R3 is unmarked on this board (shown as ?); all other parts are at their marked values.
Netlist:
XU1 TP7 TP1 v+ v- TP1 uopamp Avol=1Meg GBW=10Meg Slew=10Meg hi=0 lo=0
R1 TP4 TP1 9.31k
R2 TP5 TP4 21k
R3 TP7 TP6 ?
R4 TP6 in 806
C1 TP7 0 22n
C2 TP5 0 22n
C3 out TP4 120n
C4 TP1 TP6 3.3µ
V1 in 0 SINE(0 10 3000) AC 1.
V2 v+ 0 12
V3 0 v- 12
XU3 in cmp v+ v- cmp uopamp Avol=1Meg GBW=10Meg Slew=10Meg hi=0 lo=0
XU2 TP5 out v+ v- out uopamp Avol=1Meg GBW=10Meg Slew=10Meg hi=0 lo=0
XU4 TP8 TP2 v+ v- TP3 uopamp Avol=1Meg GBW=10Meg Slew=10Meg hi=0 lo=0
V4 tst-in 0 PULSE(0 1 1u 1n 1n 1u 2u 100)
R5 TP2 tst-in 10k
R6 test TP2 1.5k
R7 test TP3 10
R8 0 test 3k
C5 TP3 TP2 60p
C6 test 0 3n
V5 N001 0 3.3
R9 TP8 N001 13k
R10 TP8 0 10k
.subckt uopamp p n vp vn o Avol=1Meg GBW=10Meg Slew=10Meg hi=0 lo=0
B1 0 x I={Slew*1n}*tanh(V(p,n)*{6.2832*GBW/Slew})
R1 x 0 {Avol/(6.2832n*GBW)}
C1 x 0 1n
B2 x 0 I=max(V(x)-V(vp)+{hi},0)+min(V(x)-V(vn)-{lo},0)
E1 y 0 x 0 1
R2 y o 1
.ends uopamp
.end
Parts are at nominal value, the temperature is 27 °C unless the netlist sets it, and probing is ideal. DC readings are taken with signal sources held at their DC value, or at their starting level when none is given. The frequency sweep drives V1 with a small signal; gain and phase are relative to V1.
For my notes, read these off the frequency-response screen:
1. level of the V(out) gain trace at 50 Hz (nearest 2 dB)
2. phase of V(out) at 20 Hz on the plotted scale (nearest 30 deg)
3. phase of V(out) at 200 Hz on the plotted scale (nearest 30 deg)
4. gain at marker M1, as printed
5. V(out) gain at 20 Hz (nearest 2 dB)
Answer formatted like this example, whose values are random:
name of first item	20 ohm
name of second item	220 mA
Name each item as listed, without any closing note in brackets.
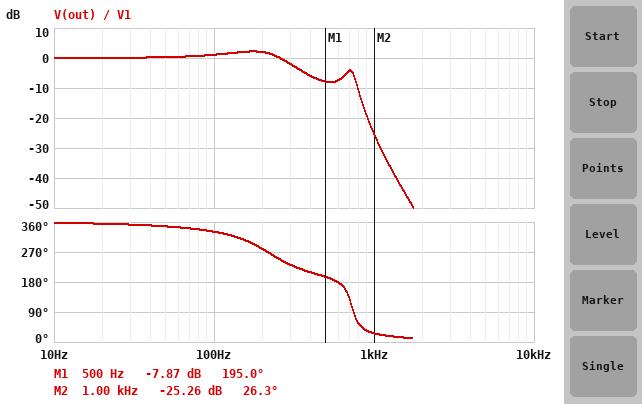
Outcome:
level of the V(out) gain trace at 50 Hz	0 dB
phase of V(out) at 20 Hz on the plotted scale	360 deg
phase of V(out) at 200 Hz on the plotted scale	270 deg
gain at marker M1, as printed	-7.87 dB
V(out) gain at 20 Hz	0 dB
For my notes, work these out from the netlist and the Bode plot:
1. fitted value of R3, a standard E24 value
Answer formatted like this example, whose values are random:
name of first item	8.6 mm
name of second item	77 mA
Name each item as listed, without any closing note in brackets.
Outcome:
fitted value of R3, a standard E24 value	820 Ω
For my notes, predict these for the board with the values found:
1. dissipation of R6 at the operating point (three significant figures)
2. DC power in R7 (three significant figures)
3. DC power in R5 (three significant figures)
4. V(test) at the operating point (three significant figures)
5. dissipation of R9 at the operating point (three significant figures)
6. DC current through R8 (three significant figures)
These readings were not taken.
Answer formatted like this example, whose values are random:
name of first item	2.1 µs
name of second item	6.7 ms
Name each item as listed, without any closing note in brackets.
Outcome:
dissipation of R6 at the operating point	30.9 µW
DC power in R7	4.81 µW
DC power in R5	206 µW
V(test) at the operating point	1.65 V
dissipation of R9 at the operating point	268 µW
DC current through R8	550 µA
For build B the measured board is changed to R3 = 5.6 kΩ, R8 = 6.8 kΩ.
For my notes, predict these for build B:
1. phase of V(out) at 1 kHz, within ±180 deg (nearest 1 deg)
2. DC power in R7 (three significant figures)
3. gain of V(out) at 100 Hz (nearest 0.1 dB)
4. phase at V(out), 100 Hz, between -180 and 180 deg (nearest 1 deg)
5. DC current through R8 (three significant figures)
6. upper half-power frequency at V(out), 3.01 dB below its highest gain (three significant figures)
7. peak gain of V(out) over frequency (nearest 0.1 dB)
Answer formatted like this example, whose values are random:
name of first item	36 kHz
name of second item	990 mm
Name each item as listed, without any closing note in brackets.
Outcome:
phase of V(out) at 1 kHz, within ±180 deg	16 deg
DC power in R7	1.49 µW
gain of V(out) at 100 Hz	2.1 dB
phase at V(out), 100 Hz, between -180 and 180 deg	-34 deg
DC current through R8	243 µA
upper half-power frequency at V(out), 3.01 dB below its highest gain	295 Hz
peak gain of V(out) over frequency	10.5 dB
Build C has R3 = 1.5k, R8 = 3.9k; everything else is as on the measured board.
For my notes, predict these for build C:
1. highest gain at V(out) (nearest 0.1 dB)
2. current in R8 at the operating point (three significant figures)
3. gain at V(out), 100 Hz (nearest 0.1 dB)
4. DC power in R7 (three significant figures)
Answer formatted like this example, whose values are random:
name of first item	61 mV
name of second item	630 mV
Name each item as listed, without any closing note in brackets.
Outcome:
highest gain at V(out)	2.7 dB
current in R8 at the operating point	423 µA
gain at V(out), 100 Hz	1.2 dB
DC power in R7	3.21 µW
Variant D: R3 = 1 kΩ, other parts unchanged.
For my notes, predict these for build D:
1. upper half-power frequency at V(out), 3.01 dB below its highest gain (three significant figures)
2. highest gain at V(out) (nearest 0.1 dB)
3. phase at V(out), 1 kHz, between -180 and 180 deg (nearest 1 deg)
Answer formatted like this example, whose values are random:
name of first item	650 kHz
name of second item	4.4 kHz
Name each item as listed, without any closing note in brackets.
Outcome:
upper half-power frequency at V(out), 3.01 dB below its highest gain	280 Hz
highest gain at V(out)	2.3 dB
phase at V(out), 1 kHz, between -180 and 180 deg	23 deg
